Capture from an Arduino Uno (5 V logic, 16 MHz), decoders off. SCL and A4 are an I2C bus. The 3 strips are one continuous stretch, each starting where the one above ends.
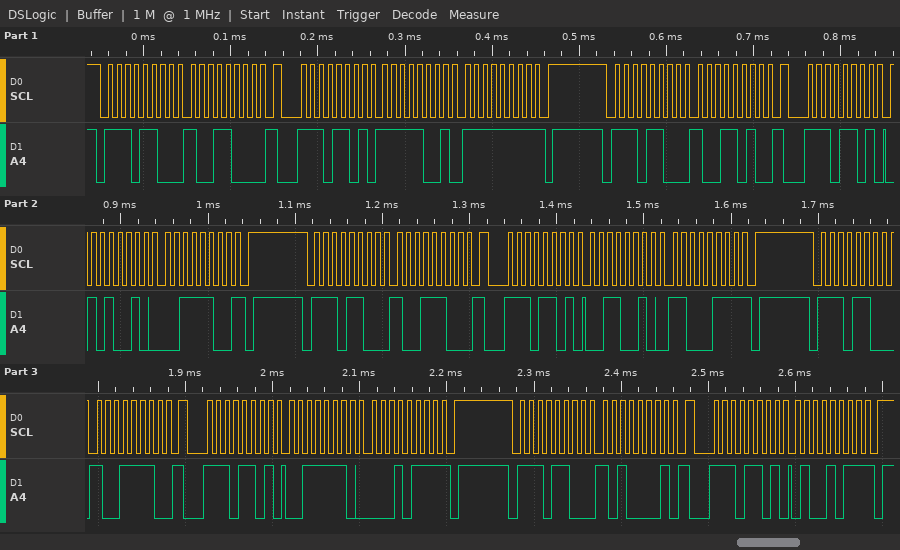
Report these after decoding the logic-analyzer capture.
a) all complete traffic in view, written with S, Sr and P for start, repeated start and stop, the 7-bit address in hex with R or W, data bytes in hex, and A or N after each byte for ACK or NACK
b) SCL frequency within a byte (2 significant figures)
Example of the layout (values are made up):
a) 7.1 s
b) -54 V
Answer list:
a) S 76W A 98 A Sr 76R A F9 A FF N P S 76W A 9A A Sr 76R A 52 A 3C N P S 76W A 9C A Sr 76R A 32 A C7 N P S 76W A 9E A Sr 76R A 3E A 17 N P S 76W A A1 A Sr 76R A 4B N P
b) 100 kHz
